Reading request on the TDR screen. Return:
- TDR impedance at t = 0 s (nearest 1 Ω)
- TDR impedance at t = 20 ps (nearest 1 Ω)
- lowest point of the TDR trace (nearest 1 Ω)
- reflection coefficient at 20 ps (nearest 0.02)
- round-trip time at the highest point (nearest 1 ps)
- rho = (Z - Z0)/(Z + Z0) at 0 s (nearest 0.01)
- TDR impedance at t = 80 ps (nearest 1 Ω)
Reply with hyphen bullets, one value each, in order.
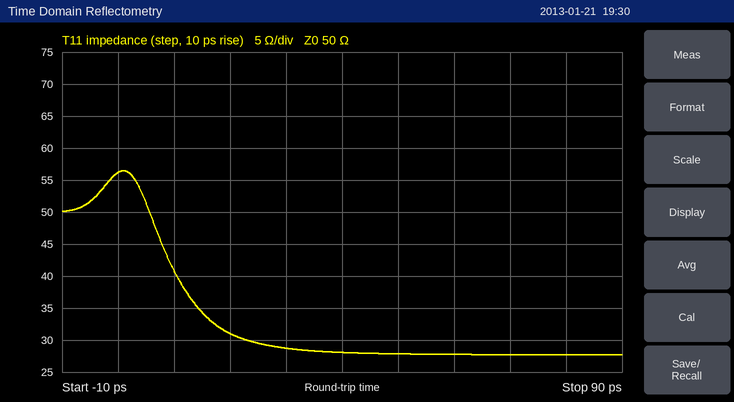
- 56 Ω
- 31 Ω
- 28 Ω
- -0.24
- 1 ps
- +0.06
- 28 Ω
